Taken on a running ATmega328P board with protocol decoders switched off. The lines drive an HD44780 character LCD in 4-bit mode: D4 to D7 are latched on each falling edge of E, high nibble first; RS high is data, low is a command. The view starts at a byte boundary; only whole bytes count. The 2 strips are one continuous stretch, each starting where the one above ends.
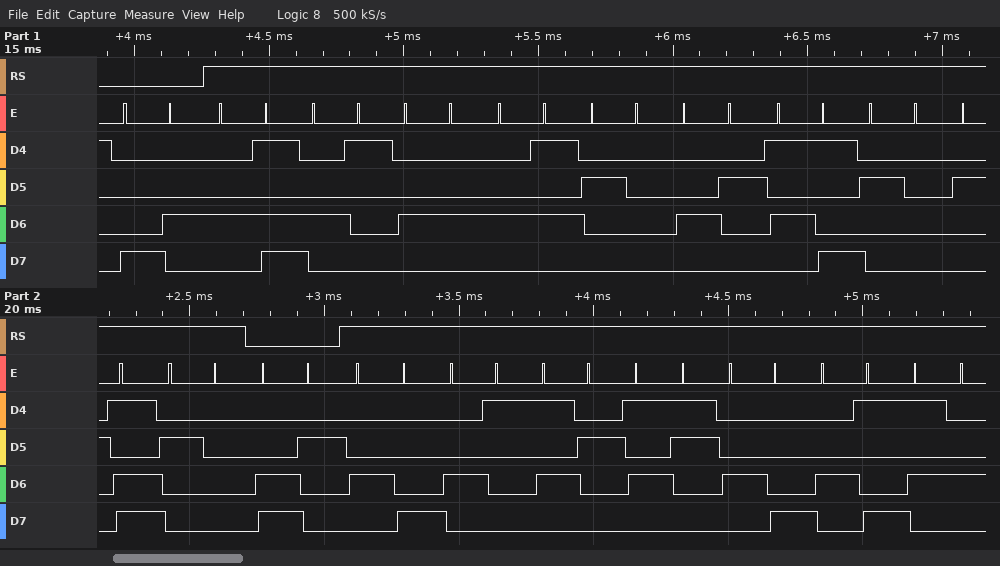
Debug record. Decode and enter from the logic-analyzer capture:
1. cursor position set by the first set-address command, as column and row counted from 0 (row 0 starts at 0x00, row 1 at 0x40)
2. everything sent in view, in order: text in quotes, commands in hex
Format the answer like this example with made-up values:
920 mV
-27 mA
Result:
column 4, row 0
0x84 "MADE BY - " 0xC2 "HARSHIT"
